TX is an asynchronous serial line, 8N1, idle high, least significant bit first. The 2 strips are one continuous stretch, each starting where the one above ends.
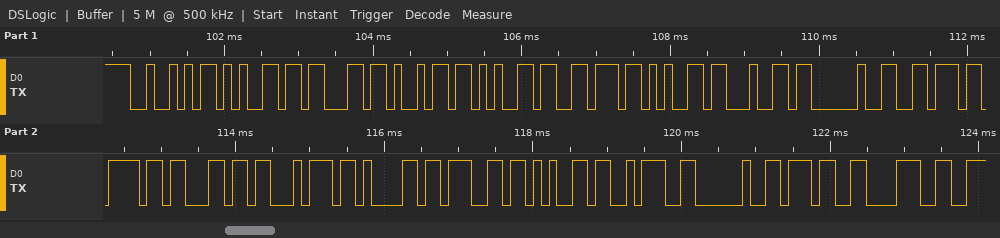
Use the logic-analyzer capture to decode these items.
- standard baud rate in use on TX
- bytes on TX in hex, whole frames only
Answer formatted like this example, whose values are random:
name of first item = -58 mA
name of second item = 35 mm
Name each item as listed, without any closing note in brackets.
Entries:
standard baud rate in use on TX = 9600 baud
bytes on TX in hex, whole frames only = 0x52 0x65 0x63 0x69 0x65 0x76 0x65 0x64 0x20 0x76 0x6F 0x6C 0x74 0x61 0x67 0x65 0x3A 0x20 0x37 0x38
